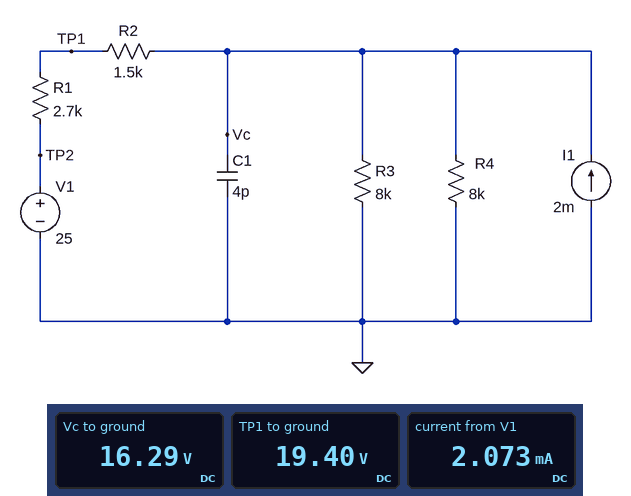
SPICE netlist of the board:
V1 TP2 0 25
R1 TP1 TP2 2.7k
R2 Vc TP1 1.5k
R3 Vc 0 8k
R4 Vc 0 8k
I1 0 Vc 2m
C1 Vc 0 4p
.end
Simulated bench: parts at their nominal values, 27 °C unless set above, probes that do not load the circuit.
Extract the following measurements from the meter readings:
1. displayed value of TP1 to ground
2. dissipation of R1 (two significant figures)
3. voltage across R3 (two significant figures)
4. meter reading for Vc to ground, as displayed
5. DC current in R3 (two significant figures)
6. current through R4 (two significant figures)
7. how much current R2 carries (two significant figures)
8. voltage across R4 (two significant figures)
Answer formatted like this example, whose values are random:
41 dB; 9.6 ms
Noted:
19.40 V; 12 mW; 16 V; 16.29 V; 2.0 mA; 2.0 mA; 2.1 mA; 16 V
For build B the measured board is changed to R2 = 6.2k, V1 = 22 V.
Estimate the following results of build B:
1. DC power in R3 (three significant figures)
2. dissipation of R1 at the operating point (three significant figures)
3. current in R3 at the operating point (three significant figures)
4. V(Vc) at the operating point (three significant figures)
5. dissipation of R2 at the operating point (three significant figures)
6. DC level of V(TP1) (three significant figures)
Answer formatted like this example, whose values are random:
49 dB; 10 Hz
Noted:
19.0 mW; 3.18 mW; 1.54 mA; 12.3 V; 7.30 mW; 19.1 V
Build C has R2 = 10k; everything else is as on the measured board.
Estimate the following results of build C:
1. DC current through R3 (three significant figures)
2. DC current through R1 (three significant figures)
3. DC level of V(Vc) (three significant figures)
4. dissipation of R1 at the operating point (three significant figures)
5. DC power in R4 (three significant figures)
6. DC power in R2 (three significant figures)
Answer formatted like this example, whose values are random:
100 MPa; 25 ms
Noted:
1.51 mA; 1.02 mA; 12.1 V; 2.80 mW; 18.2 mW; 10.4 mW
